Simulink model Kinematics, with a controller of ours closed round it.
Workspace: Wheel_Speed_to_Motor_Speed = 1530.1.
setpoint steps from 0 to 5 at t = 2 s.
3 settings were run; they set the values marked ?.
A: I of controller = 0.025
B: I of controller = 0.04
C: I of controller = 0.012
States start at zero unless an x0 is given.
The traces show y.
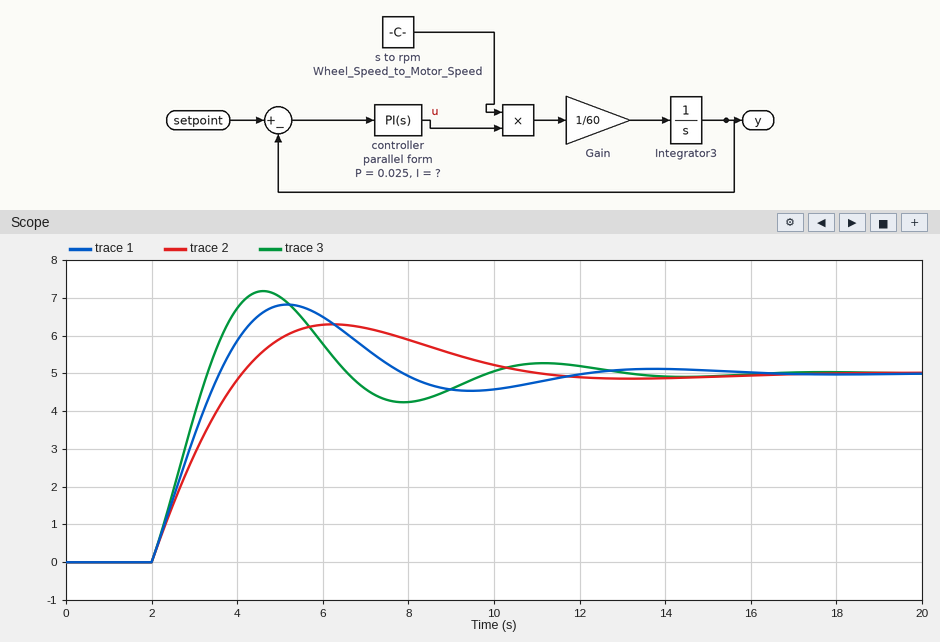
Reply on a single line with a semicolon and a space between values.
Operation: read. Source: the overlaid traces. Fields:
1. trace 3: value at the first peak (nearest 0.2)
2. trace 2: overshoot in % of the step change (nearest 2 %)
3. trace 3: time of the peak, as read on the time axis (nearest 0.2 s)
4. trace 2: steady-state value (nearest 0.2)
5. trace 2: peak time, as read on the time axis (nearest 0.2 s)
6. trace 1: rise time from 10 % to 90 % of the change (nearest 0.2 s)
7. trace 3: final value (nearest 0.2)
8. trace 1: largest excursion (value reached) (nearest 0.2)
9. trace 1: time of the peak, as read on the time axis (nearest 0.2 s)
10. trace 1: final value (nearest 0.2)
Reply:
7.2; 26 %; 4.6 s; 5.0; 6.2 s; 1.2 s; 5.0; 6.8; 5.2 s; 5.0
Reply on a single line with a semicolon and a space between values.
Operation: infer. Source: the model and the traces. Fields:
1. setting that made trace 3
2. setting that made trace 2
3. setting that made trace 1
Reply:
B; C; A
